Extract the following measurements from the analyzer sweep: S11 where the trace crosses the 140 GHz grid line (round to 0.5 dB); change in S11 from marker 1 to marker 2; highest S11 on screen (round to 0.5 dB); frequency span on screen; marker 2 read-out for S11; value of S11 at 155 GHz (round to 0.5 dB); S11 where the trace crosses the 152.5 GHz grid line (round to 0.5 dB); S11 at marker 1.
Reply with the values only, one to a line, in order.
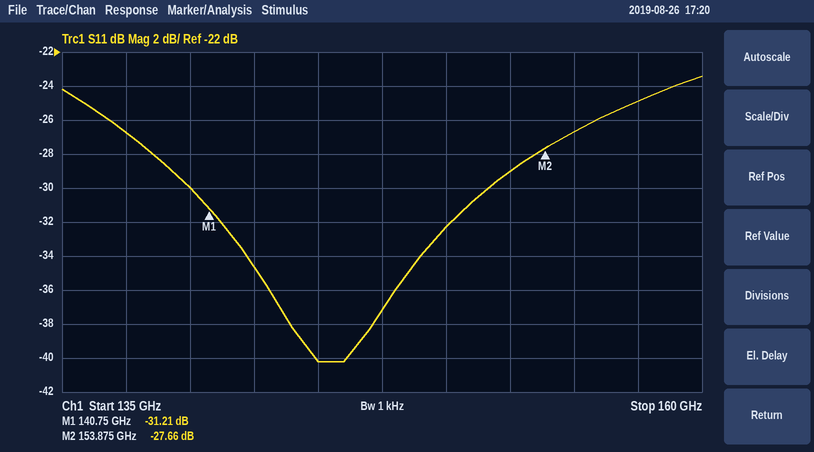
-30.0 dB
3.55 dB
-23.5 dB
25 GHz
-27.66 dB
-26.5 dB
-29.0 dB
-31.21 dB
